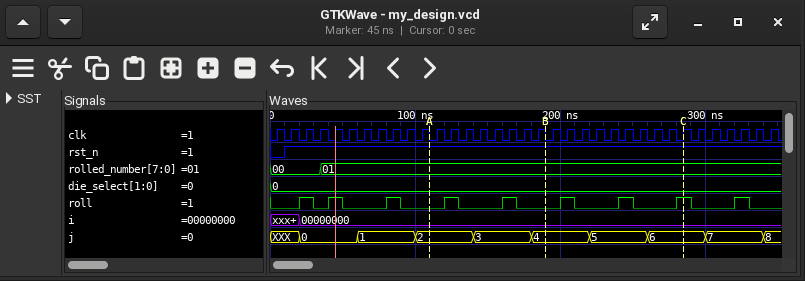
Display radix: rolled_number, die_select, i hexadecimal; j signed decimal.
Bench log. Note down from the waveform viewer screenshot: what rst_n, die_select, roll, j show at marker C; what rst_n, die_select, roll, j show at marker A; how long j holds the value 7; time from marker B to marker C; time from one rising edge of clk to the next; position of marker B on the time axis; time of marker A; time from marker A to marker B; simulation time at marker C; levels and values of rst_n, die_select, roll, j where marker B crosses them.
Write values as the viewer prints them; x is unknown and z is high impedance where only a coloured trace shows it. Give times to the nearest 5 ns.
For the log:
rst_n=1, die_select=0, roll=1, j=6
rst_n=1, die_select=0, roll=0, j=2
40 ns
95 ns
10 ns
190 ns
110 ns
80 ns
285 ns
rst_n=1, die_select=0, roll=0, j=4
